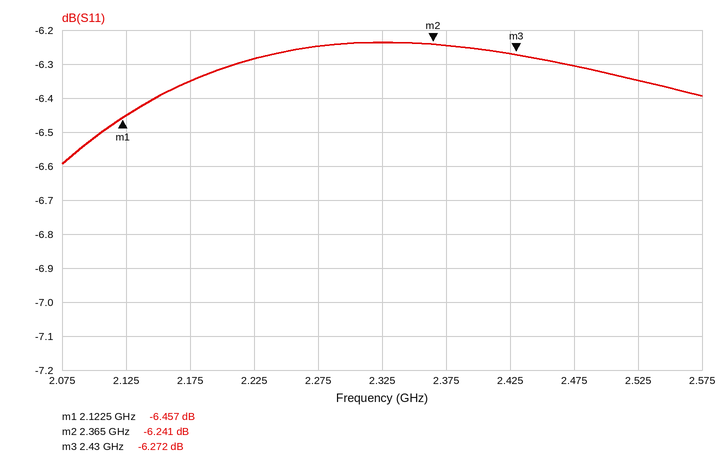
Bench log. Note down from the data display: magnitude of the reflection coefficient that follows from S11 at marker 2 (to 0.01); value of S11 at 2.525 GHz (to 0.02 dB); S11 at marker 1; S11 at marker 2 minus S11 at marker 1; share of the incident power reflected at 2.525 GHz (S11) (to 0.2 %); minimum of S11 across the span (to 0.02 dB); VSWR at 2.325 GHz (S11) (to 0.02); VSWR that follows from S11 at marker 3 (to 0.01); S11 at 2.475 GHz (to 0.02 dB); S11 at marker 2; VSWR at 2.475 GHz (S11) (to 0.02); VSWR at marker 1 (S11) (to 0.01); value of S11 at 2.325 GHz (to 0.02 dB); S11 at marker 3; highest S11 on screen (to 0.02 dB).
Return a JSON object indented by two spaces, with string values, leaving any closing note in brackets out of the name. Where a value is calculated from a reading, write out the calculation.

{
  "magnitude of the reflection coefficient that follows from S11 at marker 2": "10^(-6.241/20) ≈ 0.49",
  "value of S11 at 2.525 GHz": "-6.34 dB",
  "S11 at marker 1": "-6.457 dB",
  "S11 at marker 2 minus S11 at marker 1": "-6.241 − (-6.457) = 0.216 dB",
  "share of the incident power reflected at 2.525 GHz (S11)": "10^(-6.34/10) ≈ 23.2 %",
  "minimum of S11 across the span": "-6.60 dB",
  "VSWR at 2.325 GHz (S11)": "|Γ| = 10^(-6.24/20) = 0.4875; VSWR = (1 + 0.4875)/(1 − 0.4875) ≈ 2.90",
  "VSWR that follows from S11 at marker 3": "(1 + 0.4857)/(1 − 0.4857) ≈ 2.89",
  "S11 at 2.475 GHz": "-6.30 dB",
  "S11 at marker 2": "-6.241 dB",
  "VSWR at 2.475 GHz (S11)": "|Γ| = 10^(-6.3/20) = 0.4842; VSWR = (1 + 0.4842)/(1 − 0.4842) ≈ 2.88",
  "VSWR at marker 1 (S11)": "(1 + 0.4755)/(1 − 0.4755) ≈ 2.81",
  "value of S11 at 2.325 GHz": "-6.24 dB",
  "S11 at marker 3": "-6.272 dB",
  "highest S11 on screen": "-6.24 dB"
}
